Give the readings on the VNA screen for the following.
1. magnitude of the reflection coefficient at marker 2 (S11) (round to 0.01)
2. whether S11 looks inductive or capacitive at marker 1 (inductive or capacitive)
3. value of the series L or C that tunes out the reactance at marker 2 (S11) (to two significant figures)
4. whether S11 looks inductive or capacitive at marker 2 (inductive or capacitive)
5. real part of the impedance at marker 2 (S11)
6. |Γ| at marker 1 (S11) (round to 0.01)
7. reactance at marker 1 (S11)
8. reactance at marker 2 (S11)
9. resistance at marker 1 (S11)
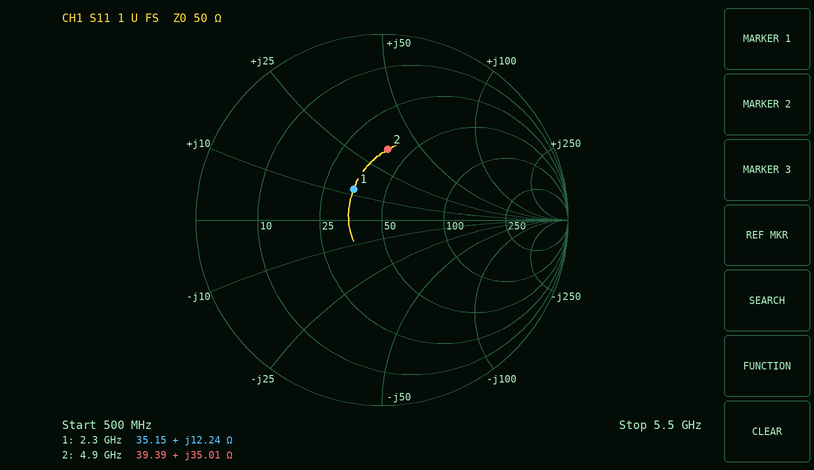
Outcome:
0.38
inductive
930 fF
inductive
39.39 Ω
0.22
+12.24 Ω
+35.01 Ω
35.15 Ω
